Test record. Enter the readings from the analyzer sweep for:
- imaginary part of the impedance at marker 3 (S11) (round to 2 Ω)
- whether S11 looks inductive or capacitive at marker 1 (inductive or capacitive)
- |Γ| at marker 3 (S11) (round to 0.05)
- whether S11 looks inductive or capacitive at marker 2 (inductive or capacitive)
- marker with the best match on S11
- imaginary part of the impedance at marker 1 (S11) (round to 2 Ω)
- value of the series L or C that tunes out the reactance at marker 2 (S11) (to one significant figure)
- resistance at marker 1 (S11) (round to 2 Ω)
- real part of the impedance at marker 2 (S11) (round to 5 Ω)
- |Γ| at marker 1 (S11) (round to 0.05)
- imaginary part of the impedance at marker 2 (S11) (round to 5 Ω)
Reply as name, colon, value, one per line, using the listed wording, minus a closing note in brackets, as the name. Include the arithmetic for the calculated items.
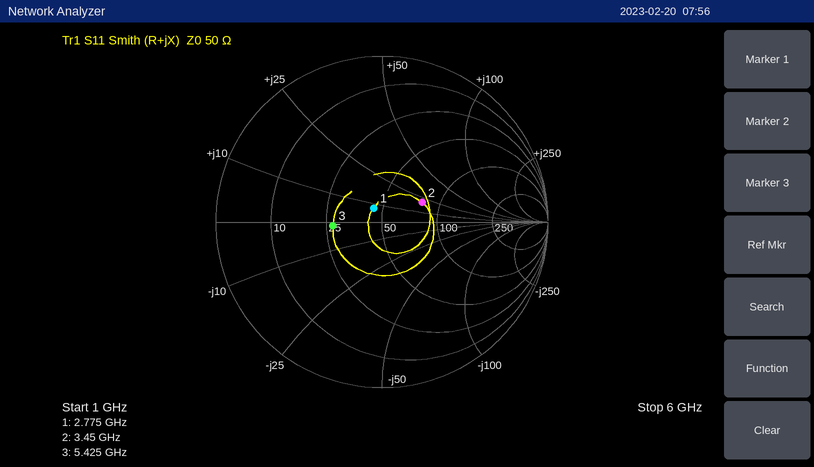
imaginary part of the impedance at marker 3 (S11): -2 Ω
whether S11 looks inductive or capacitive at marker 1: inductive
|Γ| at marker 3 (S11): 0.30
whether S11 looks inductive or capacitive at marker 2: inductive
marker with the best match on S11: marker 1
imaginary part of the impedance at marker 1 (S11): +8 Ω
value of the series L or C that tunes out the reactance at marker 2 (S11): C = 1/(2π × 3.45 GHz × 20 Ω) ≈ 2 pF
resistance at marker 1 (S11): 44 Ω
real part of the impedance at marker 2 (S11): 80 Ω
|Γ| at marker 1 (S11): 0.10
imaginary part of the impedance at marker 2 (S11): +20 Ω
